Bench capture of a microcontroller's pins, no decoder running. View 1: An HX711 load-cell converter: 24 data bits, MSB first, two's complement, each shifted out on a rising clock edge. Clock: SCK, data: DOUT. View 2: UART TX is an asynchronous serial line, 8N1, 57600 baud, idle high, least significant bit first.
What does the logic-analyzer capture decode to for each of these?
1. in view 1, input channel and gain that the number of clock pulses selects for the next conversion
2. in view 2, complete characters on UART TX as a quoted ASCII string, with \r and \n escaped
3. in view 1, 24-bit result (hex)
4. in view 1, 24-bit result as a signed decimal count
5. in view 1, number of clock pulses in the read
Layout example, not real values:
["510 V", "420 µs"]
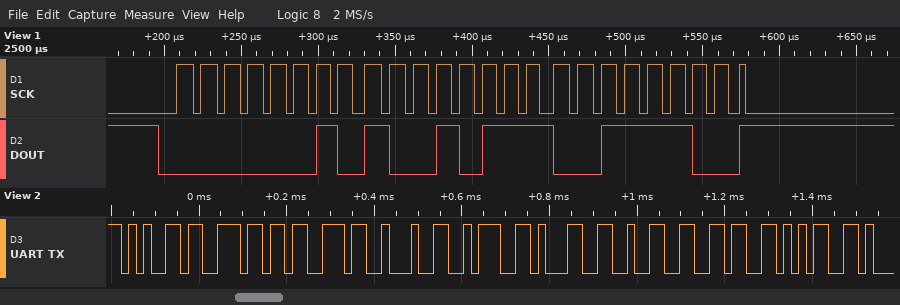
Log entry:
["channel A, gain 128", "\"ens\\\":1265\"", "0x02973C", "169788", "25"]
